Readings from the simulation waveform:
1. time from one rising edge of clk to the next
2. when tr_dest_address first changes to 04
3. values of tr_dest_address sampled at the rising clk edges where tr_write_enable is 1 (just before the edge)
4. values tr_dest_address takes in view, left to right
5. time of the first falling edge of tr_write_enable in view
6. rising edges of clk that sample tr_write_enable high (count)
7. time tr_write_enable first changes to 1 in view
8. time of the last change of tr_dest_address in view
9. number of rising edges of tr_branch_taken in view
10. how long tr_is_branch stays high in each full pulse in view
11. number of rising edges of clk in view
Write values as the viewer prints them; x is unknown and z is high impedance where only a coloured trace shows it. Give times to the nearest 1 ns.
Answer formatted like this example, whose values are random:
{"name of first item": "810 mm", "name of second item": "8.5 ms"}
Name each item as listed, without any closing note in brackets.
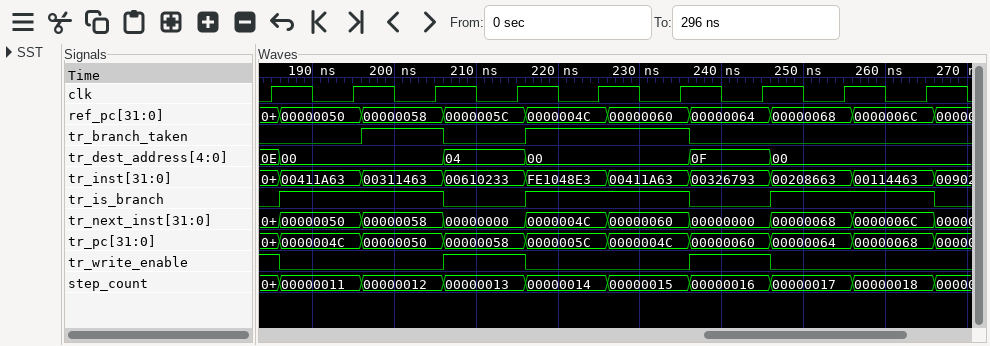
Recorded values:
{"time from one rising edge of clk to the next": "10 ns", "when tr_dest_address first changes to 04": "206 ns", "values of tr_dest_address sampled at the rising clk edges where tr_write_enable is 1": "0E, 04, 0F", "values tr_dest_address takes in view, left to right": "0E, 00, 04, 00, 0F, 00", "time of the first falling edge of tr_write_enable in view": "186 ns", "rising edges of clk that sample tr_write_enable high": "3", "time tr_write_enable first changes to 1 in view": "206 ns", "time of the last change of tr_dest_address in view": "246 ns", "number of rising edges of tr_branch_taken in view": "2", "how long tr_is_branch stays high in each full pulse in view": "20 ns, 20 ns, 20 ns", "number of rising edges of clk in view": "9"}
